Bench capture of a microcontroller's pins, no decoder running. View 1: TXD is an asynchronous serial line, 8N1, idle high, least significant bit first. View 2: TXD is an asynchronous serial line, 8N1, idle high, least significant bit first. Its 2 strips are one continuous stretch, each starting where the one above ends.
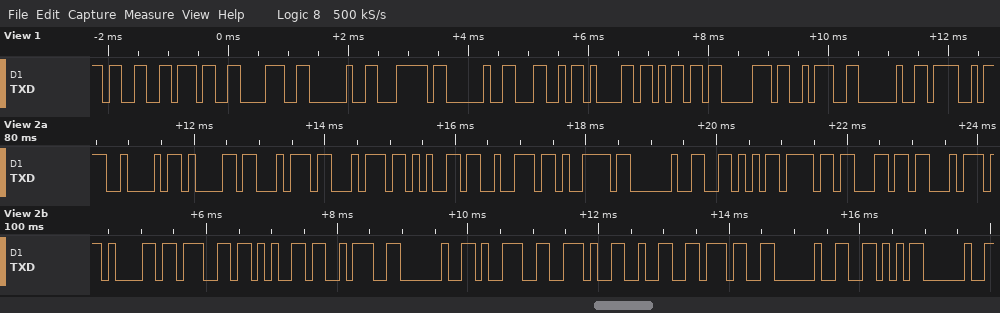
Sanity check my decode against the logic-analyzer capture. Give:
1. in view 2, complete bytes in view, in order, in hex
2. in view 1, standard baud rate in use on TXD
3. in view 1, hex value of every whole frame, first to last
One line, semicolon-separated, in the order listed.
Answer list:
42 61 74 74 65 72 79 20 56 6F 6C 74 61 67 65 3A 20 39 2E 32 37 20 56 20; 9600 baud; 33 37 38 20 7C 20 4C 61 6D 70 3A 20 4F
